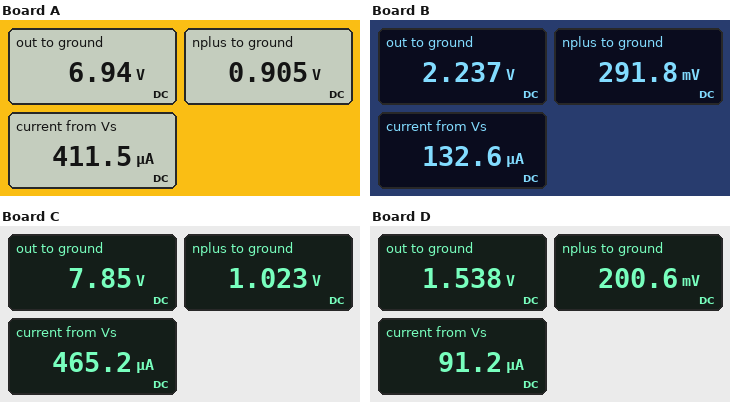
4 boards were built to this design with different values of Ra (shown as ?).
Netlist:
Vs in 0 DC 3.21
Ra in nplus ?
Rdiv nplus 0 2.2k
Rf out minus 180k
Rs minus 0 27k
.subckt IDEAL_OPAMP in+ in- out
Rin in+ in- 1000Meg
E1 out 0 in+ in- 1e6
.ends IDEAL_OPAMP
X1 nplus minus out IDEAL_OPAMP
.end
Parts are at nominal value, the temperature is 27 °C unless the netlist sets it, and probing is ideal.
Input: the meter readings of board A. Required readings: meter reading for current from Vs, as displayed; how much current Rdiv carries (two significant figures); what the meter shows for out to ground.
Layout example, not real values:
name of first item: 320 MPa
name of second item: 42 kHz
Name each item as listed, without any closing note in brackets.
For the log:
meter reading for current from Vs, as displayed: 411.5 µA
how much current Rdiv carries: 410 µA
what the meter shows for out to ground: 6.94 V
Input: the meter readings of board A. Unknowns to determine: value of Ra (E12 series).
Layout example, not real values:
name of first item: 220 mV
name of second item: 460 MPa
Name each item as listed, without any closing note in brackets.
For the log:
value of Ra: 5.6 kΩ
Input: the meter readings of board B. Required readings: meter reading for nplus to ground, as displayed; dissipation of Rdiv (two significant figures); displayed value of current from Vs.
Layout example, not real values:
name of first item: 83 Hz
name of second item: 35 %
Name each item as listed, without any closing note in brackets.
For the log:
meter reading for nplus to ground, as displayed: 291.8 mV
dissipation of Rdiv: 39 µW
displayed value of current from Vs: 132.6 µA
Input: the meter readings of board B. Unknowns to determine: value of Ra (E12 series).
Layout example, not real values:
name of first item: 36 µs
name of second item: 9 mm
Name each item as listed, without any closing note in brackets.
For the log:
value of Ra: 22 kΩ
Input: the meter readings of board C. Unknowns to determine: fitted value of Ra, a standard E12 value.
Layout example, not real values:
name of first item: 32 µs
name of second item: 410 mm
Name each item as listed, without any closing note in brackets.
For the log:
fitted value of Ra, a standard E12 value: 4.7 kΩ
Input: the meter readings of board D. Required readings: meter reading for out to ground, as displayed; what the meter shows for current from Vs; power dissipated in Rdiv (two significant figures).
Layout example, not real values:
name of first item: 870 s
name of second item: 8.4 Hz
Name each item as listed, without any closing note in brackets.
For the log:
meter reading for out to ground, as displayed: 1.538 V
what the meter shows for current from Vs: 91.2 µA
power dissipated in Rdiv: 18 µW
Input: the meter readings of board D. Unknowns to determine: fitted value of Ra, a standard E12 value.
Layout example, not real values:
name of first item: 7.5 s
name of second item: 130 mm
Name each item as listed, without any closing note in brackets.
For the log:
fitted value of Ra, a standard E12 value: 33 kΩ
